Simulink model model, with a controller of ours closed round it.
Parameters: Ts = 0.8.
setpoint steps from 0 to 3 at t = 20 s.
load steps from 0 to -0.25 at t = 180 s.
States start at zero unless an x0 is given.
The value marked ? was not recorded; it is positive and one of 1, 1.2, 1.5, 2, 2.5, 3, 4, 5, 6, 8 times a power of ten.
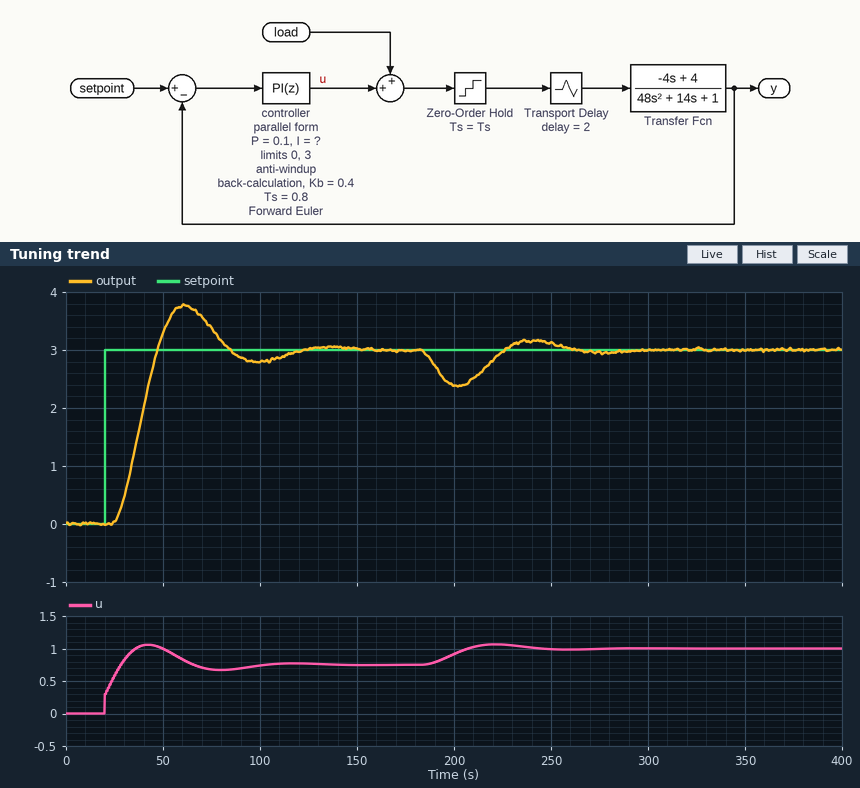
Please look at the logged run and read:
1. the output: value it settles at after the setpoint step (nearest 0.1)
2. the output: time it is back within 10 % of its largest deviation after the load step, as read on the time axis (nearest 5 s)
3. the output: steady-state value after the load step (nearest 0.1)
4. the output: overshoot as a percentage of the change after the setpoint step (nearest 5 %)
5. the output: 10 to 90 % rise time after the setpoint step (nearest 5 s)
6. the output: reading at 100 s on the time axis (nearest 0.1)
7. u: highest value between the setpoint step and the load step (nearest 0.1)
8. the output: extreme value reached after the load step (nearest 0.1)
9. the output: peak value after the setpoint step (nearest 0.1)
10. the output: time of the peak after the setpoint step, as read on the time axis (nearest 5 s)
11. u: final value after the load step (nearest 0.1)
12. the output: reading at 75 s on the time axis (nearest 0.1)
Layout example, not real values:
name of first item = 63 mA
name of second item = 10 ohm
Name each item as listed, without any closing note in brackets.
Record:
the output: value it settles at after the setpoint step = 3.0
the output: time it is back within 10 % of its largest deviation after the load step, as read on the time axis = 255 s
the output: steady-state value after the load step = 3.0
the output: overshoot as a percentage of the change after the setpoint step = 25 %
the output: 10 to 90 % rise time after the setpoint step = 15 s
the output: reading at 100 s on the time axis = 2.8
u: highest value between the setpoint step and the load step = 1.1
the output: extreme value reached after the load step = 2.4
the output: peak value after the setpoint step = 3.8
the output: time of the peak after the setpoint step, as read on the time axis = 60 s
u: final value after the load step = 1.0
the output: reading at 75 s on the time axis = 3.4
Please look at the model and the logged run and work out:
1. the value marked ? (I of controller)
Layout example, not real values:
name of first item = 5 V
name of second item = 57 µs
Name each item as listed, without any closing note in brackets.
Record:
the value marked ? = 0.02
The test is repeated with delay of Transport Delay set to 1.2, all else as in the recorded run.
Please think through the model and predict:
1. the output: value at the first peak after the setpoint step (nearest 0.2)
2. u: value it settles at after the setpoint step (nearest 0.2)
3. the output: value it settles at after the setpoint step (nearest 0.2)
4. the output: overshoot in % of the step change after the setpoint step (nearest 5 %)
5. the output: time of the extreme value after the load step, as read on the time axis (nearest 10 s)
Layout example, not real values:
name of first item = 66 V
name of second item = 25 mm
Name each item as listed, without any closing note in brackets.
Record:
the output: value at the first peak after the setpoint step = 3.6
u: value it settles at after the setpoint step = 0.8
the output: value it settles at after the setpoint step = 3.0
the output: overshoot in % of the step change after the setpoint step = 20 %
the output: time of the extreme value after the load step, as read on the time axis = 200 s
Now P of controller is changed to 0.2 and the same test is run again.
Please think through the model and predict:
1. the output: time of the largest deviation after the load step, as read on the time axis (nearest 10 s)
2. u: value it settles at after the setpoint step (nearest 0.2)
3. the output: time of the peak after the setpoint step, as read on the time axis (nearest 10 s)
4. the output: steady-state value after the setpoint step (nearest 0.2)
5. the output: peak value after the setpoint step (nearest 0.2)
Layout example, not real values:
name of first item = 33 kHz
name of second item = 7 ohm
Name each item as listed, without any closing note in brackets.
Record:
the output: time of the largest deviation after the load step, as read on the time axis = 200 s
u: value it settles at after the setpoint step = 0.8
the output: time of the peak after the setpoint step, as read on the time axis = 50 s
the output: steady-state value after the setpoint step = 3.0
the output: peak value after the setpoint step = 3.4
